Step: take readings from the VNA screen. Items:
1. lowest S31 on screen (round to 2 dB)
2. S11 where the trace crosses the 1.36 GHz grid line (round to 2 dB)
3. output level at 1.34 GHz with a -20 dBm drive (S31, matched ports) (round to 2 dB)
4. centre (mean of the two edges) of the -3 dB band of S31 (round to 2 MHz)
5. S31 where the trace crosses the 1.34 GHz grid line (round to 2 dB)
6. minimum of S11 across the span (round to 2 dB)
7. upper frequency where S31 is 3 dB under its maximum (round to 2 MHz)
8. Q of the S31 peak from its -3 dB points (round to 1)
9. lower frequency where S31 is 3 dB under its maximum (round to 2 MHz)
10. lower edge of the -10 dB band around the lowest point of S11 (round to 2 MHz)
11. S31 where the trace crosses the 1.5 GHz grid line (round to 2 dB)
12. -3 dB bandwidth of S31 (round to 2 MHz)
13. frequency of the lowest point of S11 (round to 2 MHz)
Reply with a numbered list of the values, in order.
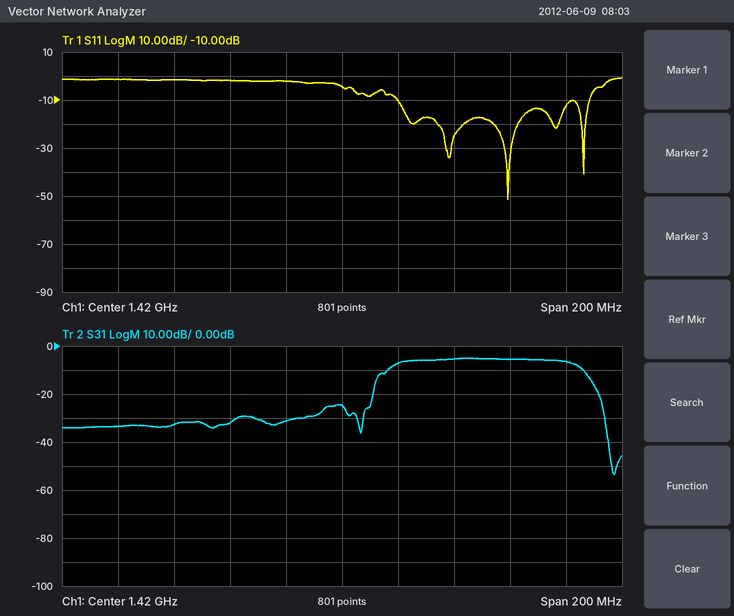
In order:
1. -54 dB
2. -2 dB
3. -54 dBm
4. 1.472 GHz
5. -34 dB
6. -52 dB
7. 1.504 GHz
8. 22
9. 1.438 GHz
10. 1.440 GHz
11. -6 dB
12. 66 MHz
13. 1.480 GHz
